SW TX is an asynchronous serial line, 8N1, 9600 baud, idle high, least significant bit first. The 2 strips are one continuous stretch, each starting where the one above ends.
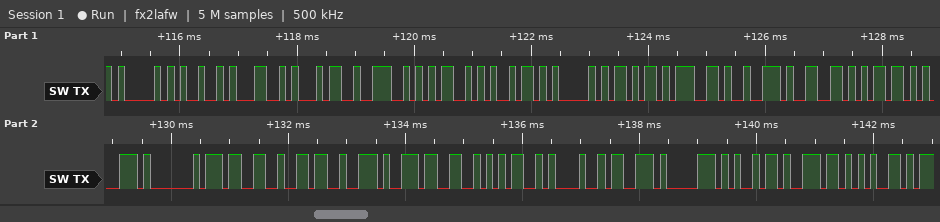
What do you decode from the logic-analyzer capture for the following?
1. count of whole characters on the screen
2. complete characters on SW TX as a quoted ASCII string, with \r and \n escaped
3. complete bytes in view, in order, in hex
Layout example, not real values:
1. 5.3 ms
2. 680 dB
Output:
1. 26
2. "AIL4NMiAkgrfmq@36.35!spine"
3. 41 49 4C 34 4E 4D 69 41 6B 67 72 66 6D 71 40 33 36 2E 33 35 21 73 70 69 6E 65
